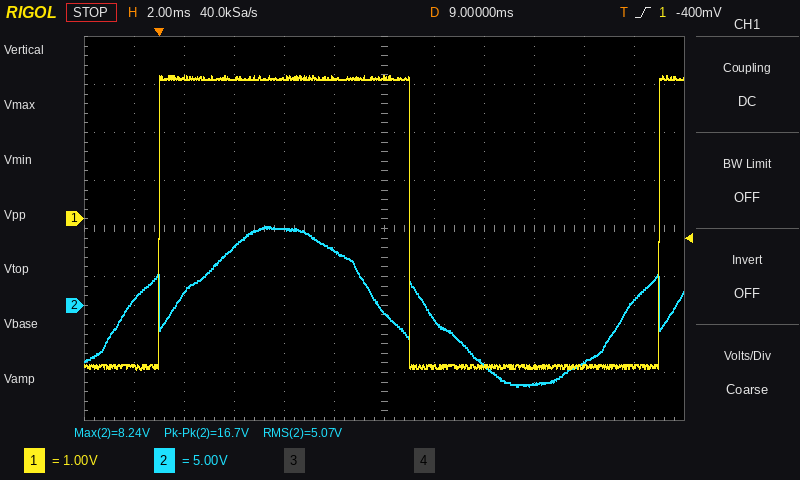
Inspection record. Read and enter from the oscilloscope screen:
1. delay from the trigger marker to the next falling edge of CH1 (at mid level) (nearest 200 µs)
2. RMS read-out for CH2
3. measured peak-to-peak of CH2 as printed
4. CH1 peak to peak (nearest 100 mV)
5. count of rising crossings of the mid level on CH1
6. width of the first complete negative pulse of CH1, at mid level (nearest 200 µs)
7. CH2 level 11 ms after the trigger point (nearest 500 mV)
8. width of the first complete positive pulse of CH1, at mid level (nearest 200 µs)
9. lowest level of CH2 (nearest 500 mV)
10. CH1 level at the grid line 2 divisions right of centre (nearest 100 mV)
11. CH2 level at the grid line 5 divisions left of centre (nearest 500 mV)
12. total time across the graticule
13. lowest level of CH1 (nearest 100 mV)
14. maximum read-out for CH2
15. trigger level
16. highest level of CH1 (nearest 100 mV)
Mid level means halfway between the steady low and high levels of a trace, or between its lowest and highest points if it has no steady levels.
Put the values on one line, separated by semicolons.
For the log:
10.0 ms; 5.07 V; 16.7 V; 6.1 V; 2; 10.0 ms; -1.5 V; 10.0 ms; -8.5 V; -3.1 V; 500 mV; 24 ms; -3.1 V; 8.24 V; -400 mV; 3.0 V
